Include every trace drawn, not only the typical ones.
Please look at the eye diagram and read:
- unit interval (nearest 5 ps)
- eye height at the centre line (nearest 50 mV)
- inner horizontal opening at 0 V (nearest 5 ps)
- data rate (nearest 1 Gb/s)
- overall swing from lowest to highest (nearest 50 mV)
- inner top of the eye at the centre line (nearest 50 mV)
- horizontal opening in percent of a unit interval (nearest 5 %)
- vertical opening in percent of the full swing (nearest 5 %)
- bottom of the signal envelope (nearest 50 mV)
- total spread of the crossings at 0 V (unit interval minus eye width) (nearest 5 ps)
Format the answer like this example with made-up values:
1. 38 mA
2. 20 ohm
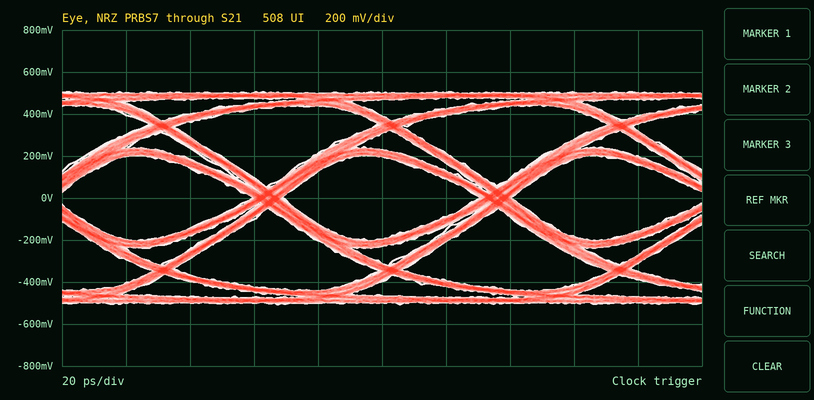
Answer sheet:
1. 70 ps
2. 400 mV
3. 60 ps
4. 14 Gb/s
5. 1.00 V
6. 200 mV
7. 85 %
8. 40 %
9. -500 mV
10. 10 ps
